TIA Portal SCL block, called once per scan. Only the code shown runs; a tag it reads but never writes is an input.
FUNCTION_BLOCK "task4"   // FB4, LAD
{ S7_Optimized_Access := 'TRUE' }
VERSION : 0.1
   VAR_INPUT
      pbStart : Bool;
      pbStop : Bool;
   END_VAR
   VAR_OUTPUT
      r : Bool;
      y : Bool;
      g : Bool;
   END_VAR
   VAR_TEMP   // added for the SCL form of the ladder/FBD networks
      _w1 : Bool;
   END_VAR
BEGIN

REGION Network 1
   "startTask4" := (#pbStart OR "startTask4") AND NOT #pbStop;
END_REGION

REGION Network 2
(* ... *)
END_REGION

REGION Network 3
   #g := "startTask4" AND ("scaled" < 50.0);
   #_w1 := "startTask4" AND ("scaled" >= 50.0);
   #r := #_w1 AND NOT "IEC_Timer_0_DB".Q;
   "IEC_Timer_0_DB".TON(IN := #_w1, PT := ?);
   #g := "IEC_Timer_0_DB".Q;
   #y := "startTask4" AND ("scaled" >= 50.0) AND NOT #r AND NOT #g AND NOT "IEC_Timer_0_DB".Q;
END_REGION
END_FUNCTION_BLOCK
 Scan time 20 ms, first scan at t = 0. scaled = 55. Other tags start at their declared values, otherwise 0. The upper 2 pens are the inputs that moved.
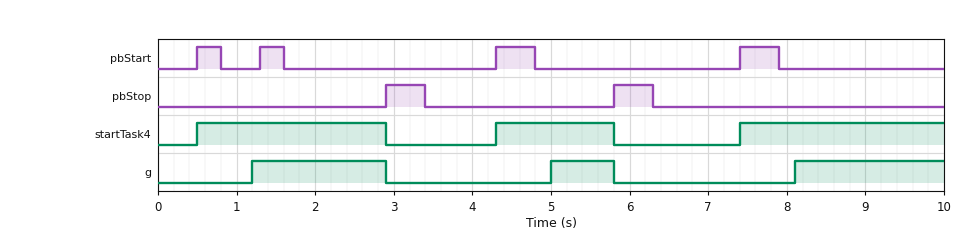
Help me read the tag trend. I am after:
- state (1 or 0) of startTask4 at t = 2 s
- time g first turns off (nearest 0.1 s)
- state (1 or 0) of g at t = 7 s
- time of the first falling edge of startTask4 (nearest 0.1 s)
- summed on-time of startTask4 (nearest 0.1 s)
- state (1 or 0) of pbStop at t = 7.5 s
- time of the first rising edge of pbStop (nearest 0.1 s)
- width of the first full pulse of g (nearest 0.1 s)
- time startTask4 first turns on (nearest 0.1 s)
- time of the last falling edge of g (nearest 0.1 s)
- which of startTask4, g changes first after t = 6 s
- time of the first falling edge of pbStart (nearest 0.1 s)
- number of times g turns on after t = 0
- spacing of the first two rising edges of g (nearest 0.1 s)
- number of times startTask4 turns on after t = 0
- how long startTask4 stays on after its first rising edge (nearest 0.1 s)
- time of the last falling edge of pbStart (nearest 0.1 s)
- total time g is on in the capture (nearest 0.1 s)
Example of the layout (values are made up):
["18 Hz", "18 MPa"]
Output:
["1", "2.9 s", "0", "2.9 s", "6.5 s", "0", "2.9 s", "1.7 s", "0.5 s", "5.8 s", "startTask4", "0.8 s", "3", "3.8 s", "3", "2.4 s", "7.9 s", "4.4 s"]
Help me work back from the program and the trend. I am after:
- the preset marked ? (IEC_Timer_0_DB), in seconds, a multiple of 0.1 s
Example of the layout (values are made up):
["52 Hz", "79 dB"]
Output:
["0.7 s"]
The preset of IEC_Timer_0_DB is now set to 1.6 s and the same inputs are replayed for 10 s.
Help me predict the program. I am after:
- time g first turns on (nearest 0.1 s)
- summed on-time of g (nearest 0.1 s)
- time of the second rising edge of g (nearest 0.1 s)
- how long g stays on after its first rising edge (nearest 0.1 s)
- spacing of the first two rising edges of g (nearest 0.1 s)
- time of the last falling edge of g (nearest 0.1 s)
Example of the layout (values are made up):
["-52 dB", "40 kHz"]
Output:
["2.1 s", "1.8 s", "9.0 s", "0.8 s", "6.9 s", "2.9 s"]
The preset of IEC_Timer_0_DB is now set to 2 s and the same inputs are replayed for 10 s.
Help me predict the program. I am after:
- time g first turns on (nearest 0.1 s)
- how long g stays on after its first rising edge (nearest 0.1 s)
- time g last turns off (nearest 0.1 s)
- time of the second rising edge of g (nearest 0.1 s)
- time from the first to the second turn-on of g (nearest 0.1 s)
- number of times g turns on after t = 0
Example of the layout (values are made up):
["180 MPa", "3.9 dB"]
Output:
["2.5 s", "0.4 s", "2.9 s", "9.4 s", "6.9 s", "2"]
